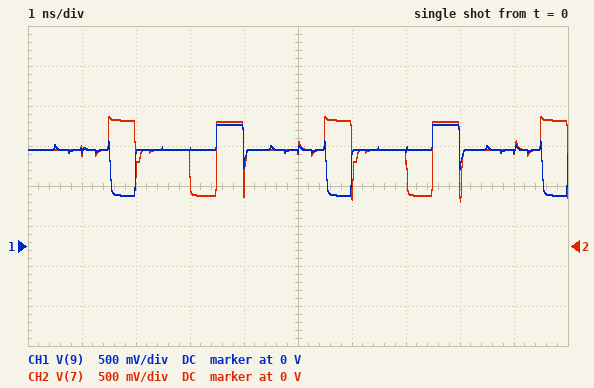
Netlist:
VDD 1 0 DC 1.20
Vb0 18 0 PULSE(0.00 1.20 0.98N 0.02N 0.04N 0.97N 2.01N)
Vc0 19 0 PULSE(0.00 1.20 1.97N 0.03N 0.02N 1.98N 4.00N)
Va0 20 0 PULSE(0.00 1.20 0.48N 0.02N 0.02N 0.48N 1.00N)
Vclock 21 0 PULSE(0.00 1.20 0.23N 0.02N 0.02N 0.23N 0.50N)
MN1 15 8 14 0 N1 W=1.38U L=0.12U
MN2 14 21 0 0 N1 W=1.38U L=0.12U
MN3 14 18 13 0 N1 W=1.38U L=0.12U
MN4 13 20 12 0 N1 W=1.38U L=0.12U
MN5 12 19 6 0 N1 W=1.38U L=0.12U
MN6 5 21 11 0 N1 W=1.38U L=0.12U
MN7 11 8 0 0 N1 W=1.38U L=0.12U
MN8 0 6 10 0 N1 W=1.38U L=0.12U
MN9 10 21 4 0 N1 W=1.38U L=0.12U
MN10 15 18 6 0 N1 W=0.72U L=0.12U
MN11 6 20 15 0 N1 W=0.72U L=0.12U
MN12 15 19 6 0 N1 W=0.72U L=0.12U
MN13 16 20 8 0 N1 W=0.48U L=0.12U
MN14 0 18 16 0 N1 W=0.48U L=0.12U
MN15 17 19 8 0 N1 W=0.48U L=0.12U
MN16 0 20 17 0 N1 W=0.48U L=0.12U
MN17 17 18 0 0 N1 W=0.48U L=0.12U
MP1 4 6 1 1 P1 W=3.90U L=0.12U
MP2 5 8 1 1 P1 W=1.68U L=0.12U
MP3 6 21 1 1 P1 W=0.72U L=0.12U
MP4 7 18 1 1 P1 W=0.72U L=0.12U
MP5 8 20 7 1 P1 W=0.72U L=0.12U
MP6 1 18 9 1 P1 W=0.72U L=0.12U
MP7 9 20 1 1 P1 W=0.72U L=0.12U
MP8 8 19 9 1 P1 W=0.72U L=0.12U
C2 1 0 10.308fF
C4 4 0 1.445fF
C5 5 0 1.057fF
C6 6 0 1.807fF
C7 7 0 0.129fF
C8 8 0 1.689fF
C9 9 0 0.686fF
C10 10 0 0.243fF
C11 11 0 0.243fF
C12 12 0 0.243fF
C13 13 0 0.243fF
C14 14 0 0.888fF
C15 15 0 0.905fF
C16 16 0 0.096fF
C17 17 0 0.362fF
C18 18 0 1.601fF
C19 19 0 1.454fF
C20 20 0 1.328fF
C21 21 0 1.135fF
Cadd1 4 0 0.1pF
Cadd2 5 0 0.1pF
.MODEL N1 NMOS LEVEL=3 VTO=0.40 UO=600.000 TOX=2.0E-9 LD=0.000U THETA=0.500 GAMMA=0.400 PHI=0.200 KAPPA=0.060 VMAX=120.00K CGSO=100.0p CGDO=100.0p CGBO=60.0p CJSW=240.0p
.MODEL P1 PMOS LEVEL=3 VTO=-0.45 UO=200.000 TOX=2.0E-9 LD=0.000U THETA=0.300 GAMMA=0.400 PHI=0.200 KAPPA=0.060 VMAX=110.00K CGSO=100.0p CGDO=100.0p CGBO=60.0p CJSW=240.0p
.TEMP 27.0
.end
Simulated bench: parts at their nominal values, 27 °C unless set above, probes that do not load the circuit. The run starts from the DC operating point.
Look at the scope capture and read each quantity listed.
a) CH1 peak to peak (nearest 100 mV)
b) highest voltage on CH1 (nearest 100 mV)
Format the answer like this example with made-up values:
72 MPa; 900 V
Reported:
900 mV; 1.5 V
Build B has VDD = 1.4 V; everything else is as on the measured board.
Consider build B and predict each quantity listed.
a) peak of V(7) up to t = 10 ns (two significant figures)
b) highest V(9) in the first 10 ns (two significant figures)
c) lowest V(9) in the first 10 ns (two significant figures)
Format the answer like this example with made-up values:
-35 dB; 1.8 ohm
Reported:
1.7 V; 1.6 V; 660 mV
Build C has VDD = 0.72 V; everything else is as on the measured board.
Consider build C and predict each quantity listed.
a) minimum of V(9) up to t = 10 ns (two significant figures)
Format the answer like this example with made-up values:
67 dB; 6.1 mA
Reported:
530 mV
